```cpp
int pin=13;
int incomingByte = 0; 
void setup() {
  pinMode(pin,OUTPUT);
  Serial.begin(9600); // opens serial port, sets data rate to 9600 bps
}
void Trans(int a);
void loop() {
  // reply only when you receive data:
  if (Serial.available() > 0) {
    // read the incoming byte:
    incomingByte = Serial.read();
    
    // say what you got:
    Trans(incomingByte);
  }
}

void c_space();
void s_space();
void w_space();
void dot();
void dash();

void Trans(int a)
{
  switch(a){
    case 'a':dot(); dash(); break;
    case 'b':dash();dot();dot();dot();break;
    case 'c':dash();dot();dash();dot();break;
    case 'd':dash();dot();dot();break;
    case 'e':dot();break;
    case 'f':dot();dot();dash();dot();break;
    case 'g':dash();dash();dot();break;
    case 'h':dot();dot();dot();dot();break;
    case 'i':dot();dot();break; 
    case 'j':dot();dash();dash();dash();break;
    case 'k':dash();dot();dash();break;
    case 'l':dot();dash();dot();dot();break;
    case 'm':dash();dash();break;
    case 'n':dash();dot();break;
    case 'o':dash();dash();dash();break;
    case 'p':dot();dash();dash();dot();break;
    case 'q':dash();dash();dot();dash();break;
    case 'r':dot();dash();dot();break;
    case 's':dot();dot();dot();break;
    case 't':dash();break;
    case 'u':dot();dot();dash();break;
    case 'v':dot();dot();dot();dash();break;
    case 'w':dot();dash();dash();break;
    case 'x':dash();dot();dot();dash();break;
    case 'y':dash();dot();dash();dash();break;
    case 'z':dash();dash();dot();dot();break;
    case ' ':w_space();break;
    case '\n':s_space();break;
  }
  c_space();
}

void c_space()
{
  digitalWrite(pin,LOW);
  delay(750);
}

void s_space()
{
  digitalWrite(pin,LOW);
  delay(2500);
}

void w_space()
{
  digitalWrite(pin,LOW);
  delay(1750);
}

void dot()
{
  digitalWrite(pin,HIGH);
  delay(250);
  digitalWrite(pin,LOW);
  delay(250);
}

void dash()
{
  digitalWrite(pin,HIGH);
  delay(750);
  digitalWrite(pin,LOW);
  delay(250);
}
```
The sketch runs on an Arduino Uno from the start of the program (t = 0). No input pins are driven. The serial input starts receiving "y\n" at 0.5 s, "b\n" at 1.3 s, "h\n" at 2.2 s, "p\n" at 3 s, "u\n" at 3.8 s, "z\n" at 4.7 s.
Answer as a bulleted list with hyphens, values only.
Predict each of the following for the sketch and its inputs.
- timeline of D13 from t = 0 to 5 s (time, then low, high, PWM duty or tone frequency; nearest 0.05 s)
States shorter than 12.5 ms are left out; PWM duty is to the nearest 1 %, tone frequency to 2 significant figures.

- 0 s low; 0.5 s high; 1.25 s low; 1.5 s high; 1.75 s low; 2 s high; 2.75 s low; 3 s high; 3.75 s low
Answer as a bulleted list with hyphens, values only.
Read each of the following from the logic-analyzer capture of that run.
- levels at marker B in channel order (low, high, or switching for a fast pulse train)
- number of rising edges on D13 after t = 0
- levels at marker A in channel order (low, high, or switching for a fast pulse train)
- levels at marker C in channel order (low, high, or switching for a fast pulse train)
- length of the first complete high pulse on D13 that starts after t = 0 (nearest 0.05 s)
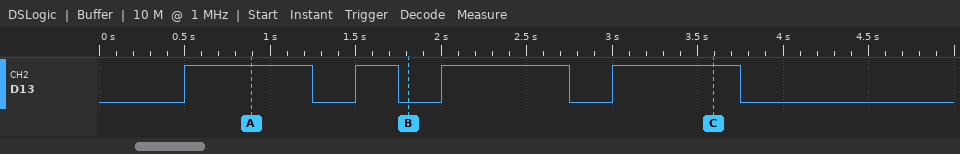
- D13 low
- 4
- D13 high
- D13 high
- 0.75 s
